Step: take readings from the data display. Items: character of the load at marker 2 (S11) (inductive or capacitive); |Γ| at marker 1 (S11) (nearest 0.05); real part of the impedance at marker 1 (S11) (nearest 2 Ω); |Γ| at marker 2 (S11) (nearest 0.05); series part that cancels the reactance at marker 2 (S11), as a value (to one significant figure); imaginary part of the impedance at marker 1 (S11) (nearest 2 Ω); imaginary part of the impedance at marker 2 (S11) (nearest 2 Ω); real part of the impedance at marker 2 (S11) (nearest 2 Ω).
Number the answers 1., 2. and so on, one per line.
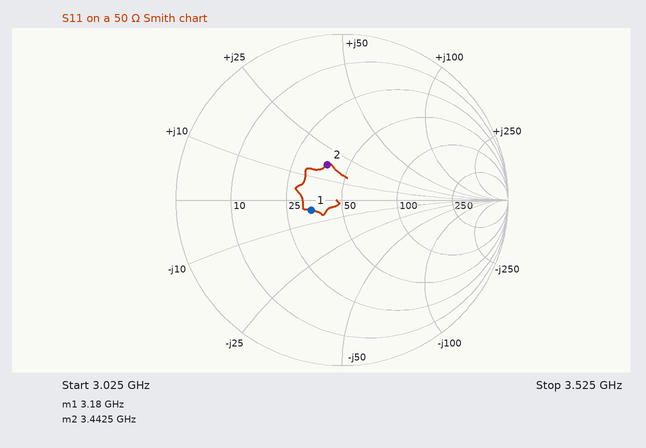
1. inductive
2. 0.20
3. 34 Ω
4. 0.25
5. 3 pF
6. -4 Ω
7. +18 Ω
8. 38 Ω
